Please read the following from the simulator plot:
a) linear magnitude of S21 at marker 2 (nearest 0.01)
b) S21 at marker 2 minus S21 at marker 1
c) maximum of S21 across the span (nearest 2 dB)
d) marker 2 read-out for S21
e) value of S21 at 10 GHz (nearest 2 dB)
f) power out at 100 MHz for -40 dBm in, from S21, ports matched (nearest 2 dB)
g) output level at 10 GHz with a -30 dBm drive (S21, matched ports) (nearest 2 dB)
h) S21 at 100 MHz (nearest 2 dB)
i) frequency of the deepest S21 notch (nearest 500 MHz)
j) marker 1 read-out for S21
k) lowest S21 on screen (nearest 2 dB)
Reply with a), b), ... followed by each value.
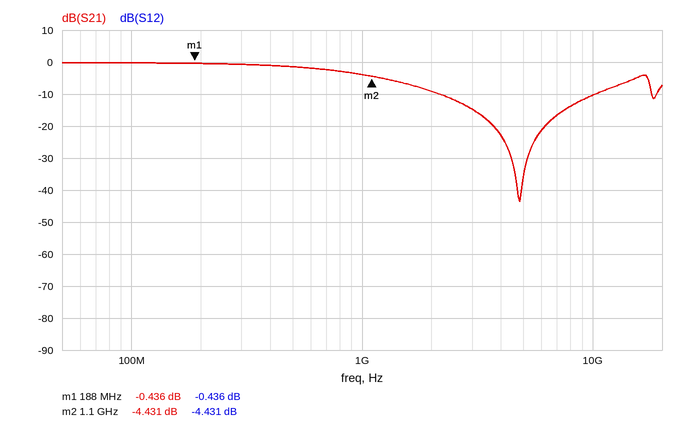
a) 0.60
b) -3.995 dB
c) 0 dB
d) -4.431 dB
e) -10 dB
f) -40 dBm
g) -40 dBm
h) 0 dB
i) 5.0 GHz
j) -0.436 dB
k) -44 dB
